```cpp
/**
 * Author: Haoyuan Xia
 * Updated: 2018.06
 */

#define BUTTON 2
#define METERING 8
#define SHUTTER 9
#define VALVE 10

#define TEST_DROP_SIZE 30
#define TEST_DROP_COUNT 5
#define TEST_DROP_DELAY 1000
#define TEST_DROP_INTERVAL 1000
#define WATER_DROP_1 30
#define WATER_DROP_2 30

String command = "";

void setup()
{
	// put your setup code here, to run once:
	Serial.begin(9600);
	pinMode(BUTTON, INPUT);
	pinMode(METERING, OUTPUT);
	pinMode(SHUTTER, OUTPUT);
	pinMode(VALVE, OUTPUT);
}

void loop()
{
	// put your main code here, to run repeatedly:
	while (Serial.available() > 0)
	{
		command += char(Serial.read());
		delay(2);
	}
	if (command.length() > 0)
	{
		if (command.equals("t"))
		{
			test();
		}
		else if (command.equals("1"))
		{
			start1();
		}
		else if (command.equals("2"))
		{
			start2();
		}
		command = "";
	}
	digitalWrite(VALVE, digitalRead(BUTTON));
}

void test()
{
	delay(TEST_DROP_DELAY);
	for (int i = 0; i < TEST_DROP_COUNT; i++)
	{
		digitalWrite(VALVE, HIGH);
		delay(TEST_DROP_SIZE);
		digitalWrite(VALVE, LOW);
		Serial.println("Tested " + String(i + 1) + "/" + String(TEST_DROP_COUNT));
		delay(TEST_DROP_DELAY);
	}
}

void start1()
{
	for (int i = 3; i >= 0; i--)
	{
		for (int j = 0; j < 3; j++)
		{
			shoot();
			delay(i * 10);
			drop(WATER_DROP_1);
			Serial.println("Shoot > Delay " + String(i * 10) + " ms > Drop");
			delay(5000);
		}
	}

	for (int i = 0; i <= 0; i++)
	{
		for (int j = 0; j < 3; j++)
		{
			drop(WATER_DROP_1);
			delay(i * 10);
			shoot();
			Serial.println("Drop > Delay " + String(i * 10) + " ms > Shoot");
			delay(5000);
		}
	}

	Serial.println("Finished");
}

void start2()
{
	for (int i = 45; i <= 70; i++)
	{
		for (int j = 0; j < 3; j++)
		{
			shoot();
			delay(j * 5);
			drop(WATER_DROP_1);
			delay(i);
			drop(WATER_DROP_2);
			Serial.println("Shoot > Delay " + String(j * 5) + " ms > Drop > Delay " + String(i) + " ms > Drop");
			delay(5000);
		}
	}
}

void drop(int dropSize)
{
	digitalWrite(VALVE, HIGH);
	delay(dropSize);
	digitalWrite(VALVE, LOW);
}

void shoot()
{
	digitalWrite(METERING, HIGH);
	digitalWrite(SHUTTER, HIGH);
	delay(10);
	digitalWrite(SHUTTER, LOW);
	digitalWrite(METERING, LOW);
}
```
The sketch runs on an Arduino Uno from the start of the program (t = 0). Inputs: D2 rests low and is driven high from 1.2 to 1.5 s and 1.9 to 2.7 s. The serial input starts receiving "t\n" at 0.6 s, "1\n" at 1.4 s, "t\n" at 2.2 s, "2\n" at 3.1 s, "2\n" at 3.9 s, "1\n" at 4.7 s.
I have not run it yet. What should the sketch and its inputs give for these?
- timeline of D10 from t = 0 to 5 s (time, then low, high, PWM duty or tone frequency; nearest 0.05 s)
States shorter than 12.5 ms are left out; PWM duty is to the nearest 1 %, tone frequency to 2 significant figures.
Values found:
0 s low; 1.2 s high; 1.5 s low; 1.9 s high; 2.7 s low
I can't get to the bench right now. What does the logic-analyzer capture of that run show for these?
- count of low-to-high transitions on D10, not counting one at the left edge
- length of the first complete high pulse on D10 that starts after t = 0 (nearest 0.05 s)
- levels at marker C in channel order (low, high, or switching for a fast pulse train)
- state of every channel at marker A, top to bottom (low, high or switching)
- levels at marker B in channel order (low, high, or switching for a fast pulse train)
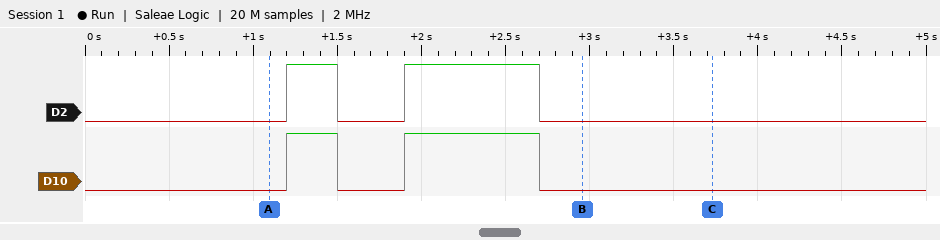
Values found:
2
0.30 s
D2 low, D10 low
D2 low, D10 low
D2 low, D10 low
